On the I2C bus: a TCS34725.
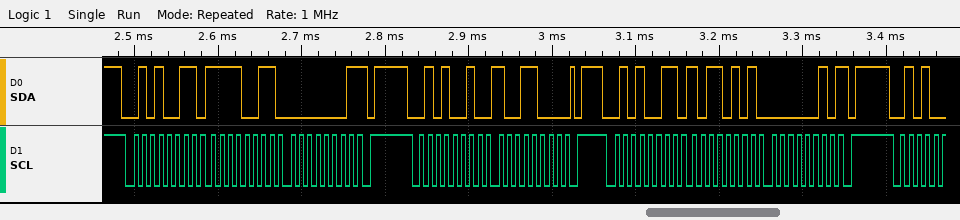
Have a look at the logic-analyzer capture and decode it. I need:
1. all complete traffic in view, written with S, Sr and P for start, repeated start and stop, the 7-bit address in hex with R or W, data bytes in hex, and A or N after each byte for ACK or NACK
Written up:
S 29R A F3 A 01 N P S 29W A 98 A P S 29R A B5 A 02 N P
